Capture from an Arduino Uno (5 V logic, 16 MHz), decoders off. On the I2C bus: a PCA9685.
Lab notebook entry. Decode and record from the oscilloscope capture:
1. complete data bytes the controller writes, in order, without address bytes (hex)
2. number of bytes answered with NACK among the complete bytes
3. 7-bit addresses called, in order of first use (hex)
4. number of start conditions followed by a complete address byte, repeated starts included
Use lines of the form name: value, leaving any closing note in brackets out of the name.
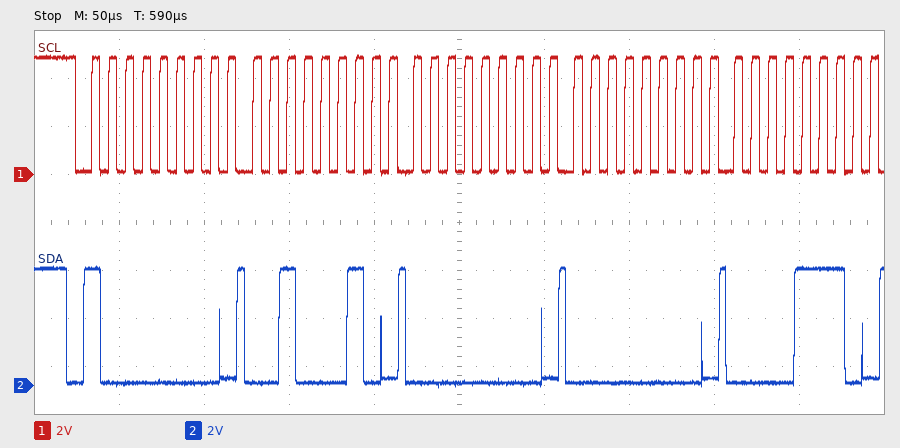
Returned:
complete data bytes the controller writes, in order, without address bytes: 22 00 00 0E
number of bytes answered with NACK among the complete bytes: 0
7-bit addresses called, in order of first use: 0x40
number of start conditions followed by a complete address byte, repeated starts included: 1
